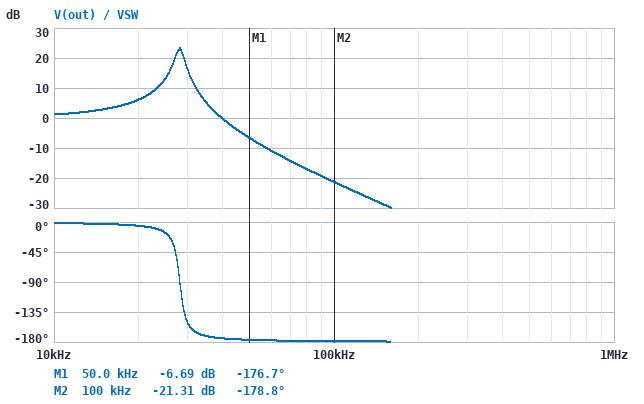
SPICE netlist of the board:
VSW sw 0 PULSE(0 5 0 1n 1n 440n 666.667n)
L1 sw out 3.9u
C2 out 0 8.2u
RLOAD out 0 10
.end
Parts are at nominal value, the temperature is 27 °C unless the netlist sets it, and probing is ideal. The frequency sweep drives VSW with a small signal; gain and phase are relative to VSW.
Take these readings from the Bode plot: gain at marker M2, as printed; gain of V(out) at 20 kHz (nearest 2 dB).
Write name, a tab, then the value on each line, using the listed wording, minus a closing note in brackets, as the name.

gain at marker M2, as printed	-21.31 dB
gain of V(out) at 20 kHz	6 dB
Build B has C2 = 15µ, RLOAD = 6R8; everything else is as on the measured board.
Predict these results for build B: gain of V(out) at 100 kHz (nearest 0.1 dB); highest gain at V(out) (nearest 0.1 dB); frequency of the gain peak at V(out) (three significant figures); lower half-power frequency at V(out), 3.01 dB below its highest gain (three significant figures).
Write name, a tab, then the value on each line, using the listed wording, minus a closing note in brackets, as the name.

gain of V(out) at 100 kHz	-26.9 dB
highest gain at V(out)	22.5 dB
frequency of the gain peak at V(out)	20.8 kHz
lower half-power frequency at V(out), 3.01 dB below its highest gain	20.0 kHz
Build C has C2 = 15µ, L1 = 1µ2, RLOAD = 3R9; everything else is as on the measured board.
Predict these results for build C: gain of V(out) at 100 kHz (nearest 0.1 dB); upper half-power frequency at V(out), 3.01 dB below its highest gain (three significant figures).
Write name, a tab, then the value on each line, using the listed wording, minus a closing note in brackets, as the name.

gain of V(out) at 100 kHz	-15.7 dB
upper half-power frequency at V(out), 3.01 dB below its highest gain	38.8 kHz
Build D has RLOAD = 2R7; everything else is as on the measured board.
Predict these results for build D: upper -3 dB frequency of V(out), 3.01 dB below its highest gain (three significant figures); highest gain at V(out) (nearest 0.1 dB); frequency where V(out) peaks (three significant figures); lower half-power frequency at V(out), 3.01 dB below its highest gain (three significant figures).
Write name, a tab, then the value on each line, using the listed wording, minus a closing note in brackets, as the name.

upper -3 dB frequency of V(out), 3.01 dB below its highest gain	31.1 kHz
highest gain at V(out)	11.9 dB
frequency where V(out) peaks	27.7 kHz
lower half-power frequency at V(out), 3.01 dB below its highest gain	23.8 kHz
